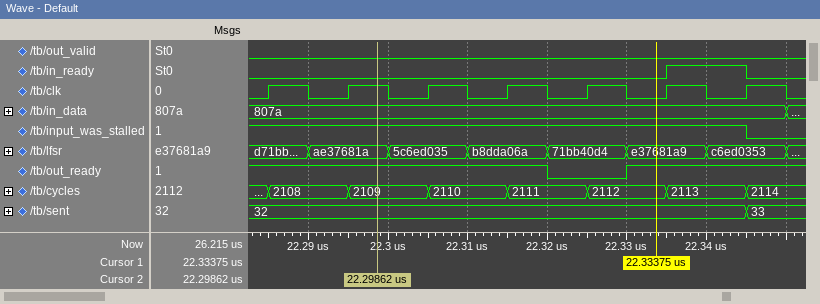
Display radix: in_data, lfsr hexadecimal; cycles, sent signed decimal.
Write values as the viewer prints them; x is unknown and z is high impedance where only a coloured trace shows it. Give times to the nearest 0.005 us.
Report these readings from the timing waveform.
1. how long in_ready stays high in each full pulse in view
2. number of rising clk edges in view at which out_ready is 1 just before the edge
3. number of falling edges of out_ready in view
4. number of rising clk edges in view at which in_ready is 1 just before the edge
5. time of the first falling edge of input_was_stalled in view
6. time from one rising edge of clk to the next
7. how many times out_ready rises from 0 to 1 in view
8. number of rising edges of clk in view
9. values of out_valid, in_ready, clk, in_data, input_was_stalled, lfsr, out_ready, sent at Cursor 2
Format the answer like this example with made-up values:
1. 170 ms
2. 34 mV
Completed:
1. 0.01 us
2. 6
3. 1
4. 1
5. 22.345 us
6. 0.01 us
7. 1
8. 7
9. out_valid=0, in_ready=0, clk=1, in_data=807a, input_was_stalled=1, lfsr=ae37681a, out_ready=1, sent=32
